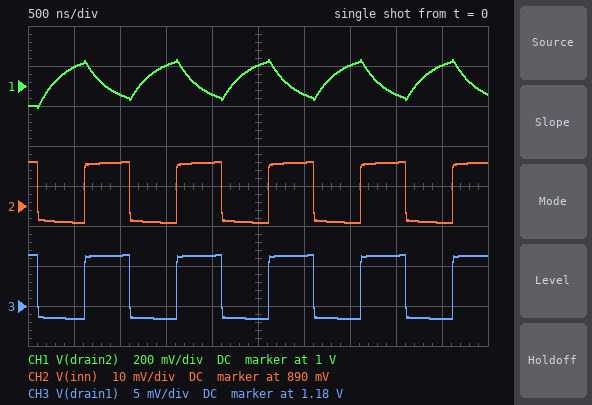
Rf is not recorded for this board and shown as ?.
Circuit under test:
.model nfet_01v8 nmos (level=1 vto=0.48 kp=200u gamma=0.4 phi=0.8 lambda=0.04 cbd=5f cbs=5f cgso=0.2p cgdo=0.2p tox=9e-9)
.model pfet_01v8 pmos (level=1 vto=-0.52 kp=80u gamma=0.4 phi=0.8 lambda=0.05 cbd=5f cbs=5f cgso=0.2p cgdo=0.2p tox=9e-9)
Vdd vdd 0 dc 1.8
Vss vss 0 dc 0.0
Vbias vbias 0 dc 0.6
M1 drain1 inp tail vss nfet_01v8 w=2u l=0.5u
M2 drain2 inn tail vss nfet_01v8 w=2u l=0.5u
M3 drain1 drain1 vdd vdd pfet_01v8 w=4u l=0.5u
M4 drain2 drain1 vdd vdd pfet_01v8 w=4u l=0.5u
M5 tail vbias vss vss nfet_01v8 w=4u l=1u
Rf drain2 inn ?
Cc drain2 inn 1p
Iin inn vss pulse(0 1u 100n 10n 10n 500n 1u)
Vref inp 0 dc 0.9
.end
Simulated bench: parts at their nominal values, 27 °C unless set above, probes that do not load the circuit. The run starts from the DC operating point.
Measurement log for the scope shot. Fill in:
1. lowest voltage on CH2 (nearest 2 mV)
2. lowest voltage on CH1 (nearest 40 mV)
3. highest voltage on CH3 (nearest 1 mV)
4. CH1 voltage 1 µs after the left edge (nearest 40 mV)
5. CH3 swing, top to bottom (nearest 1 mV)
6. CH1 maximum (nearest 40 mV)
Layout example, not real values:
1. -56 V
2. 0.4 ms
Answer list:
1. 886 mV
2. 880 mV
3. 1.186 V
4. 960 mV
5. 8 mV
6. 1.12 V
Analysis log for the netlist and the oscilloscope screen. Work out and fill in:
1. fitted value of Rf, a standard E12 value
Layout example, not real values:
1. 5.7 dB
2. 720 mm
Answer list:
1. 270 kΩ
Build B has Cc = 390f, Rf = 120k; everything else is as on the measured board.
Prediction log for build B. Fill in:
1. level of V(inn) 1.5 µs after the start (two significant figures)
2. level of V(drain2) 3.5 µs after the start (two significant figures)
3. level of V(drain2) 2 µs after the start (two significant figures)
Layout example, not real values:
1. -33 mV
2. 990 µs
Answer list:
1. 890 mV
2. 1.0 V
3. 900 mV
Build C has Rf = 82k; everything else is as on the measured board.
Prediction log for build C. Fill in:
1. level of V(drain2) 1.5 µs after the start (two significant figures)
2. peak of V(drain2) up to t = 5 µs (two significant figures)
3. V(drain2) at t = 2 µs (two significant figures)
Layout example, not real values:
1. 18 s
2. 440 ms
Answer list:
1. 970 mV
2. 980 mV
3. 900 mV
